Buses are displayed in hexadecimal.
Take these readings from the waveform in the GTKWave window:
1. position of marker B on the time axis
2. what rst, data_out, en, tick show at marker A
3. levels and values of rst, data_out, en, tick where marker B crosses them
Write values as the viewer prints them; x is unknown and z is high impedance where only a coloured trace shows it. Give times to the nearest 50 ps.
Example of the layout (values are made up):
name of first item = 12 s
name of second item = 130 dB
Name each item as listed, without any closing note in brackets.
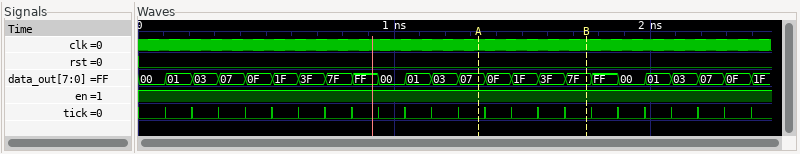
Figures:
position of marker B on the time axis = 1750 ps
what rst, data_out, en, tick show at marker A = rst=0, data_out=07, en=1, tick=0
levels and values of rst, data_out, en, tick where marker B crosses them = rst=0, data_out=7F, en=1, tick=0
